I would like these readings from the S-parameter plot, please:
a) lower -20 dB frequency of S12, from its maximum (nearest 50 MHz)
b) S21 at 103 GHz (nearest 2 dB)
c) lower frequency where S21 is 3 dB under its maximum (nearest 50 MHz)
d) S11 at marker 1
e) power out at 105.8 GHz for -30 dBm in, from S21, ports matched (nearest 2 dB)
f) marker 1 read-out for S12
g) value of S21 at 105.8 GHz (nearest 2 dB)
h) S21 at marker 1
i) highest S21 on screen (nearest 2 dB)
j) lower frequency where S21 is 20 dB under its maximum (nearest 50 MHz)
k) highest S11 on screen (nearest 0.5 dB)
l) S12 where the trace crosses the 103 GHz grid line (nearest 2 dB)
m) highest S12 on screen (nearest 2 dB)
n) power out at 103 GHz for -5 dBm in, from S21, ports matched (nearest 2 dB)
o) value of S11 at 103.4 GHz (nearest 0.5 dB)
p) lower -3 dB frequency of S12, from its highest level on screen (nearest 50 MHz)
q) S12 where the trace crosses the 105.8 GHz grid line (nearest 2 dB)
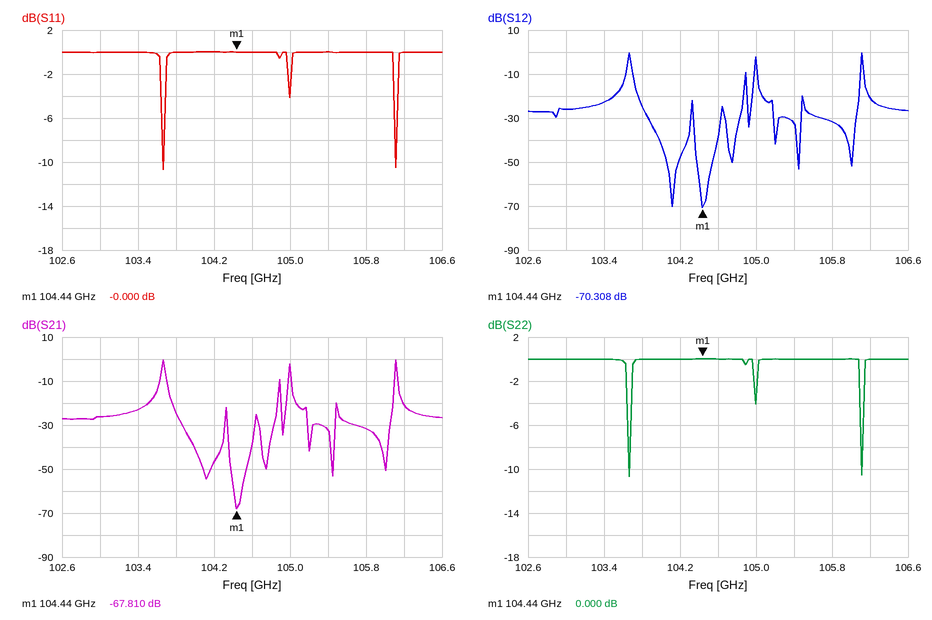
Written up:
103.50 GHz
-26 dB
103.65 GHz
-0.000 dB
-62 dBm
-70.308 dB
-32 dB
-67.810 dB
0 dB
103.50 GHz
0.0 dB
-26 dB
0 dB
-32 dBm
0.0 dB
103.65 GHz
-32 dB
